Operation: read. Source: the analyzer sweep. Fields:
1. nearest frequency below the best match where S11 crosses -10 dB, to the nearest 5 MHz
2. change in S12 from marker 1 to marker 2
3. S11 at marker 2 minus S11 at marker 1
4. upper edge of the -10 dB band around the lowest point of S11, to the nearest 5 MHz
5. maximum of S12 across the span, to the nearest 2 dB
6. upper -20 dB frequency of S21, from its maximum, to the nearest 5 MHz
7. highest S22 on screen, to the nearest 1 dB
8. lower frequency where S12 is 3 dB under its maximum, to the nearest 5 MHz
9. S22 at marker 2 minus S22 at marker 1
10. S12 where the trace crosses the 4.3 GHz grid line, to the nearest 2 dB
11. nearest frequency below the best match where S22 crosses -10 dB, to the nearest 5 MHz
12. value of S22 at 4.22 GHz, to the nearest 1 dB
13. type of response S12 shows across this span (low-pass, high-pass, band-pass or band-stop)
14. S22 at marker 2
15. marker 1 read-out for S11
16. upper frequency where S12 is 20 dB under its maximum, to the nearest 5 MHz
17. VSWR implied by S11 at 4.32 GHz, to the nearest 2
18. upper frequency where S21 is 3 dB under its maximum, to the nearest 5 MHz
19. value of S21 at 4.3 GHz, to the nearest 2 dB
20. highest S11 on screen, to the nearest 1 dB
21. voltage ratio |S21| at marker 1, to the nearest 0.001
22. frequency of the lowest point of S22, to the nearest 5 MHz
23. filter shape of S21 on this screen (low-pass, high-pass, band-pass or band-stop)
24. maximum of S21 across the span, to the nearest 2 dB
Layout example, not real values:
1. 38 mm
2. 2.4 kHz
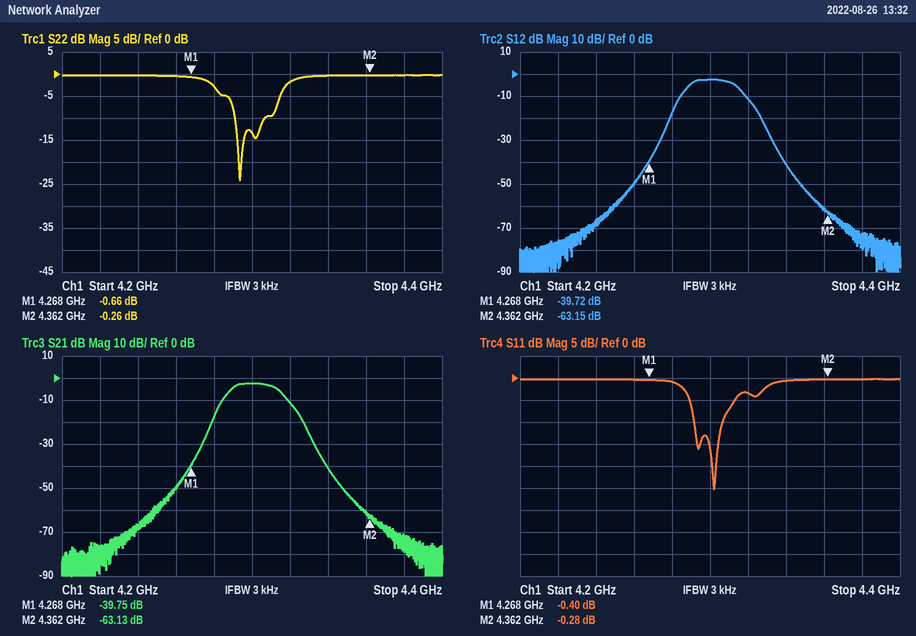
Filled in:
1. 4.290 GHz
2. -23.43 dB
3. 0.12 dB
4. 4.305 GHz
5. -2 dB
6. 4.330 GHz
7. 0 dB
8. 4.290 GHz
9. 0.40 dB
10. -2 dB
11. 4.290 GHz
12. 0 dB
13. band-pass
14. -0.26 dB
15. -0.40 dB
16. 4.330 GHz
17. 6
18. 4.315 GHz
19. -2 dB
20. 0 dB
21. 0.010
22. 4.295 GHz
23. band-pass
24. -2 dB
